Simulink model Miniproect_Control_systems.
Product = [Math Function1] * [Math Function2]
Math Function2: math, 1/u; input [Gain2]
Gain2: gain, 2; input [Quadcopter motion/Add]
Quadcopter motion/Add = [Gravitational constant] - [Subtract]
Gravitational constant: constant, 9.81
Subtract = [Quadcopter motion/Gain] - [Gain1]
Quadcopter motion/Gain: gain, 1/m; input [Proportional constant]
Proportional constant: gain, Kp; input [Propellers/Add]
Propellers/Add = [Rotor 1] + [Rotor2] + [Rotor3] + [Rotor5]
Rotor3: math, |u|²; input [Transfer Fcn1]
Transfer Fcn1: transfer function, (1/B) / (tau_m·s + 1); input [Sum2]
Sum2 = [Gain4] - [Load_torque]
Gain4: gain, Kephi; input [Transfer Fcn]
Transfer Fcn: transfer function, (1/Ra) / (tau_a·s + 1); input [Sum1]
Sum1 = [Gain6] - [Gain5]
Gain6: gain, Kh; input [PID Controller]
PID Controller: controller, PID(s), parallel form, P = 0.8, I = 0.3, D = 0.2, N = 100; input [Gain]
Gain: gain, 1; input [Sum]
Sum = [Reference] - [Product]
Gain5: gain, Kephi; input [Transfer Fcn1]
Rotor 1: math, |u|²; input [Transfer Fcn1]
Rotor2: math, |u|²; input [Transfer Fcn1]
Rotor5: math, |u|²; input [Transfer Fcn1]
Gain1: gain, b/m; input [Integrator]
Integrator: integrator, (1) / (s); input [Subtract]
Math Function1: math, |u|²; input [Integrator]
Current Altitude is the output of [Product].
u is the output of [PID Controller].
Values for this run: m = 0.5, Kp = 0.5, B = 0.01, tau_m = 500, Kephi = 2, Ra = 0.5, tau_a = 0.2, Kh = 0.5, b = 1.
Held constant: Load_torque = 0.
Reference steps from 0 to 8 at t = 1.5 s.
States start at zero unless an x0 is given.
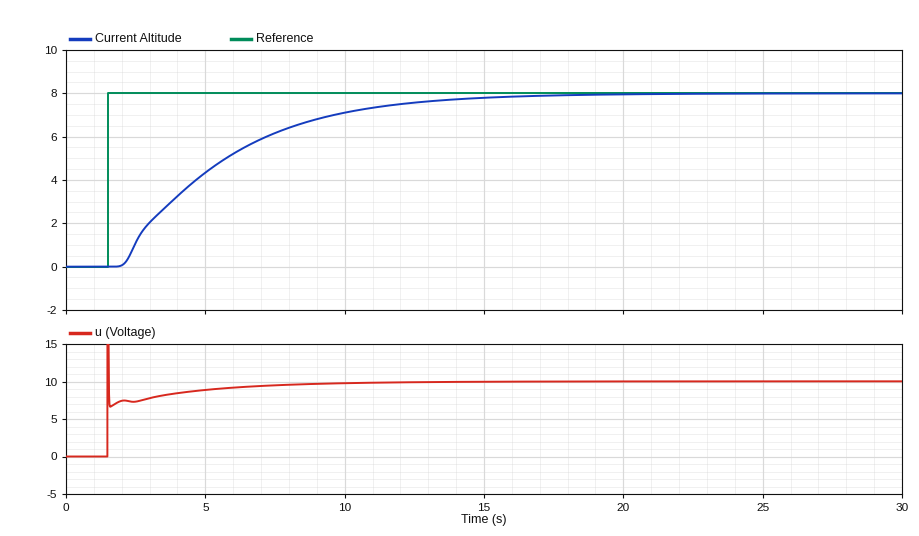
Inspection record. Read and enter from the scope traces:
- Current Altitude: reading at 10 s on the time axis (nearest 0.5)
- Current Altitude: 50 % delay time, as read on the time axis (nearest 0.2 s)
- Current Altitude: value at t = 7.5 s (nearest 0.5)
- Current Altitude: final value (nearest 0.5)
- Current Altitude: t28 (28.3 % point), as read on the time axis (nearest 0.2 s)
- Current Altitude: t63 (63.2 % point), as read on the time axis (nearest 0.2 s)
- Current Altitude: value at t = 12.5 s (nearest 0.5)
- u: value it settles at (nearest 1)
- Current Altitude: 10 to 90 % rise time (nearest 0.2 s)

7.0
4.6 s
6.0
8.0
3.2 s
5.8 s
7.5
10
8.0 s
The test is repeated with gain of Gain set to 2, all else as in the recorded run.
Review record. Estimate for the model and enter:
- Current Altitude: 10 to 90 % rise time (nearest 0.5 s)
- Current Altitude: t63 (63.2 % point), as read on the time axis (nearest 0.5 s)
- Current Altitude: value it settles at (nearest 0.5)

5.5 s
2.0 s
8.0
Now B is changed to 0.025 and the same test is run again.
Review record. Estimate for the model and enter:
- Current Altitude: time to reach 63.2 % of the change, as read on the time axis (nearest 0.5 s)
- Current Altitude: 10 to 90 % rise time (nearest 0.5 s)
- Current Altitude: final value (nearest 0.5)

5.5 s
6.0 s
8.0
